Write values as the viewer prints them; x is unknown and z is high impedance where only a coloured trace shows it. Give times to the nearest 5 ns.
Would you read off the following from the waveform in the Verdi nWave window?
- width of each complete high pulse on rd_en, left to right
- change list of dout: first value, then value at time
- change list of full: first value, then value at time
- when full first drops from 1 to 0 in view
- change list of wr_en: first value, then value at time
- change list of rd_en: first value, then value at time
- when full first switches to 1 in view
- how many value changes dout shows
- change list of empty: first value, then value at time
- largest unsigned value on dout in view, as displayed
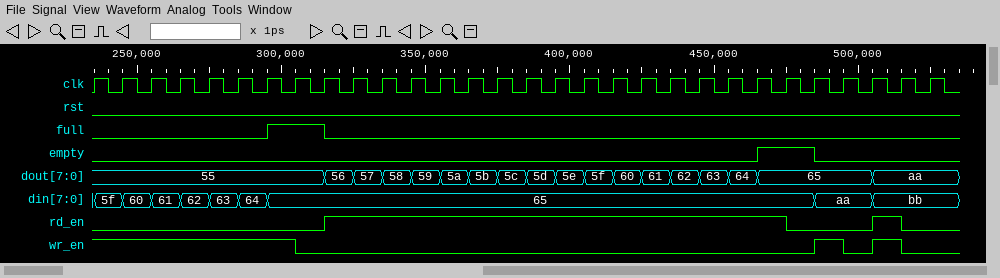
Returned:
160 ns, 10 ns
55, 56 at 315 ns, 57 at 325 ns, 58 at 335 ns, 59 at 345 ns, 5a at 355 ns, 5b at 365 ns, 5c at 375 ns, 5d at 385 ns, 5e at 395 ns, 5f at 405 ns, 60 at 415 ns, 61 at 425 ns, 62 at 435 ns, 63 at 445 ns, 64 at 455 ns, 65 at 465 ns, aa at 505 ns
0, 1 at 295 ns, 0 at 315 ns
315 ns
1, 0 at 305 ns, 1 at 485 ns, 0 at 495 ns, 1 at 505 ns, 0 at 515 ns
0, 1 at 315 ns, 0 at 475 ns, 1 at 505 ns, 0 at 515 ns
295 ns
17
0, 1 at 465 ns, 0 at 485 ns
aa
